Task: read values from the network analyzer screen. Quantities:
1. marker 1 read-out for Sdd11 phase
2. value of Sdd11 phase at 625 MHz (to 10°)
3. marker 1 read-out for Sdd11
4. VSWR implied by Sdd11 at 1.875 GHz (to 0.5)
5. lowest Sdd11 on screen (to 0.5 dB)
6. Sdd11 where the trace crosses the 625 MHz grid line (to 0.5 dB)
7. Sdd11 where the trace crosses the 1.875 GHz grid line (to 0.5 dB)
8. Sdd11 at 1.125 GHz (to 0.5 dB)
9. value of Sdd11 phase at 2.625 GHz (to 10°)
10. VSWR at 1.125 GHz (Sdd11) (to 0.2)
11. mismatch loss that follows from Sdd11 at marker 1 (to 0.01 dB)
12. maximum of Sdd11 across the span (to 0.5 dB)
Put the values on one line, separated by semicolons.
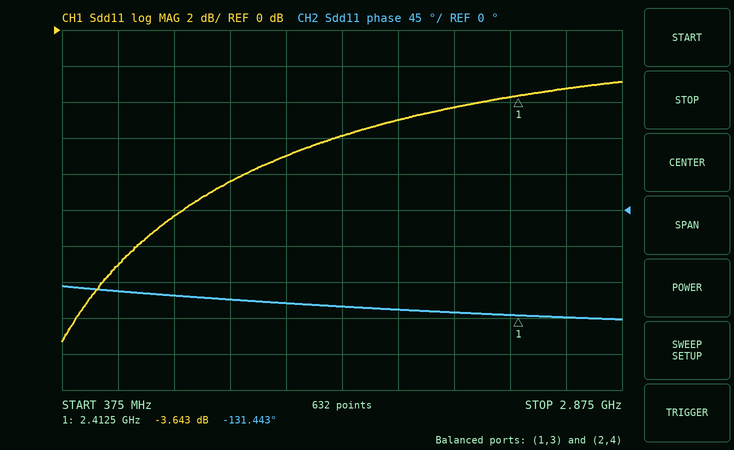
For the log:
-131.443°; -100°; -3.643 dB; 3.5; -17.5 dB; -13.0 dB; -5.0 dB; -8.5 dB; -130°; 2.2; 2.46 dB; -3.0 dB
